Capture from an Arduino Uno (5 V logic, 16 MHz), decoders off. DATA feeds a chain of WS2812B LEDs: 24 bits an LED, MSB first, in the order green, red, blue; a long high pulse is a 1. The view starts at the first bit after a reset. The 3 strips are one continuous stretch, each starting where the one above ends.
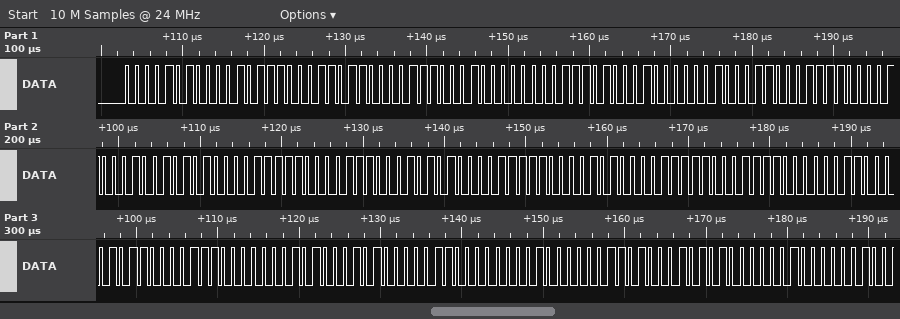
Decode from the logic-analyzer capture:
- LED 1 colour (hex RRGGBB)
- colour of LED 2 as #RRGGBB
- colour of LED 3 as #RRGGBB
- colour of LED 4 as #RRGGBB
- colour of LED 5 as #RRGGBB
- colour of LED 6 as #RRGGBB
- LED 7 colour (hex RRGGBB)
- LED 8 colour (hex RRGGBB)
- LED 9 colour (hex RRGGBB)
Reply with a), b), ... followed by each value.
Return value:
a) #170A1B
b) #200E1D
c) #23101E
d) #2A111F
e) #2A0E1F
f) #1F0A1E
g) #16061C
h) #140518
i) #0D0415
